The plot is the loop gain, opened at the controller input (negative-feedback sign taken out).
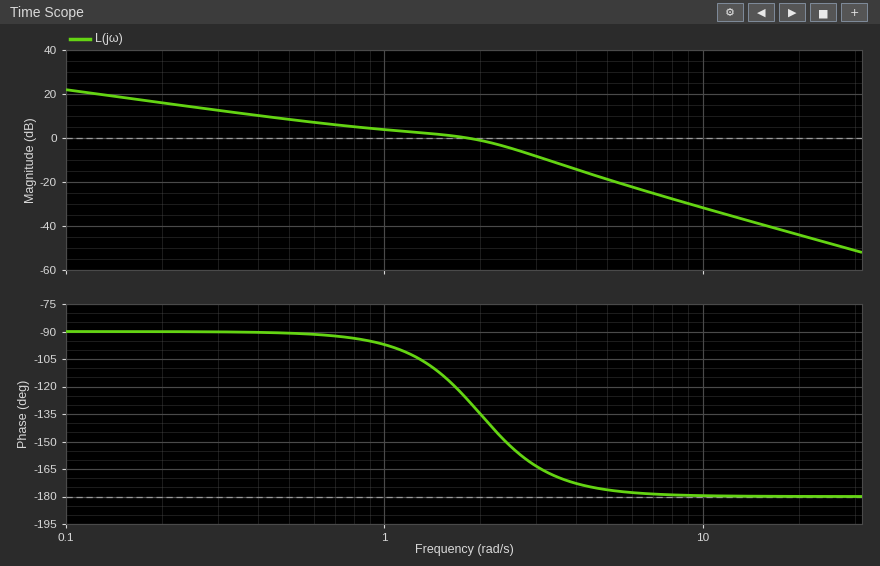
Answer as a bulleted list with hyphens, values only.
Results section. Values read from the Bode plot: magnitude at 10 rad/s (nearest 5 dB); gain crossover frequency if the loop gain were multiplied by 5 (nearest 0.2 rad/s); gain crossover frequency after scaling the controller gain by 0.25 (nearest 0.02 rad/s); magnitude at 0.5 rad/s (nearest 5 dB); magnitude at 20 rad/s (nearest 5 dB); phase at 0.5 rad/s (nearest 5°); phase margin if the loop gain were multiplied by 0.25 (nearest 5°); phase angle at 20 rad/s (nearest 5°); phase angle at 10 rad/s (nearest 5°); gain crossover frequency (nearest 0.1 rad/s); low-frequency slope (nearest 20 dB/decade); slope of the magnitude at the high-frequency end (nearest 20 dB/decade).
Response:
- -30 dB
- 4.0 rad/s
- 0.32 rad/s
- 10 dB
- -45 dB
- -90°
- 90°
- -180°
- -180°
- 1.8 rad/s
- -20 dB/decade
- -40 dB/decade
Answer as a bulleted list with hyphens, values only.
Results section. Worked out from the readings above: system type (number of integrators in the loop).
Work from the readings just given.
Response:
- 1
